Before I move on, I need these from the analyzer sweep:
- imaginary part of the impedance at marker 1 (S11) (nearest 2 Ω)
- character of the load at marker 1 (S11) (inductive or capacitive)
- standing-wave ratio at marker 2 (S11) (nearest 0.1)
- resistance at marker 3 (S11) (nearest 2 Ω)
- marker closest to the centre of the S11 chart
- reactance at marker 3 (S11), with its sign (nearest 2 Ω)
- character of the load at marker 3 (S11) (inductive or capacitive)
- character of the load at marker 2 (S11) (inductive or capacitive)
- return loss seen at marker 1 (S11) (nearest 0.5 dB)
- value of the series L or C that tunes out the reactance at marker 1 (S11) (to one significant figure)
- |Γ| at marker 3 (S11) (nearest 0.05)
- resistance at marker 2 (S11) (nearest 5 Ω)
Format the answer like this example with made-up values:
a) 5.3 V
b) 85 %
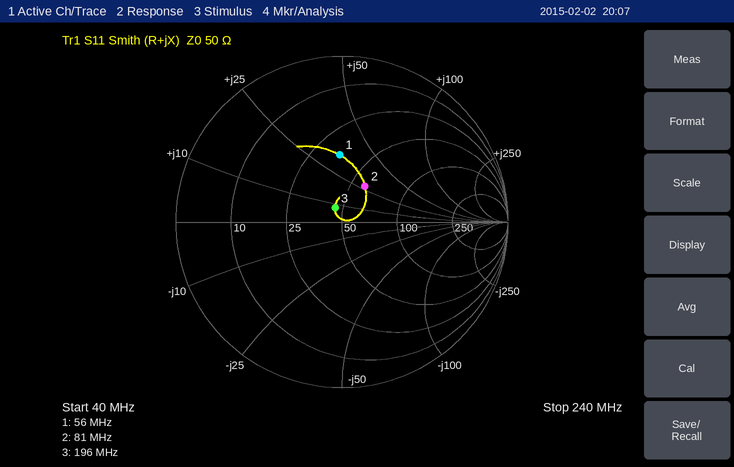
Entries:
a) +34 Ω
b) inductive
c) 1.7
d) 46 Ω
e) marker 3
f) +8 Ω
g) inductive
h) inductive
i) 8.0 dB
j) 80 pF
k) 0.10
l) 60 Ω
